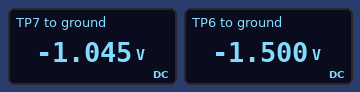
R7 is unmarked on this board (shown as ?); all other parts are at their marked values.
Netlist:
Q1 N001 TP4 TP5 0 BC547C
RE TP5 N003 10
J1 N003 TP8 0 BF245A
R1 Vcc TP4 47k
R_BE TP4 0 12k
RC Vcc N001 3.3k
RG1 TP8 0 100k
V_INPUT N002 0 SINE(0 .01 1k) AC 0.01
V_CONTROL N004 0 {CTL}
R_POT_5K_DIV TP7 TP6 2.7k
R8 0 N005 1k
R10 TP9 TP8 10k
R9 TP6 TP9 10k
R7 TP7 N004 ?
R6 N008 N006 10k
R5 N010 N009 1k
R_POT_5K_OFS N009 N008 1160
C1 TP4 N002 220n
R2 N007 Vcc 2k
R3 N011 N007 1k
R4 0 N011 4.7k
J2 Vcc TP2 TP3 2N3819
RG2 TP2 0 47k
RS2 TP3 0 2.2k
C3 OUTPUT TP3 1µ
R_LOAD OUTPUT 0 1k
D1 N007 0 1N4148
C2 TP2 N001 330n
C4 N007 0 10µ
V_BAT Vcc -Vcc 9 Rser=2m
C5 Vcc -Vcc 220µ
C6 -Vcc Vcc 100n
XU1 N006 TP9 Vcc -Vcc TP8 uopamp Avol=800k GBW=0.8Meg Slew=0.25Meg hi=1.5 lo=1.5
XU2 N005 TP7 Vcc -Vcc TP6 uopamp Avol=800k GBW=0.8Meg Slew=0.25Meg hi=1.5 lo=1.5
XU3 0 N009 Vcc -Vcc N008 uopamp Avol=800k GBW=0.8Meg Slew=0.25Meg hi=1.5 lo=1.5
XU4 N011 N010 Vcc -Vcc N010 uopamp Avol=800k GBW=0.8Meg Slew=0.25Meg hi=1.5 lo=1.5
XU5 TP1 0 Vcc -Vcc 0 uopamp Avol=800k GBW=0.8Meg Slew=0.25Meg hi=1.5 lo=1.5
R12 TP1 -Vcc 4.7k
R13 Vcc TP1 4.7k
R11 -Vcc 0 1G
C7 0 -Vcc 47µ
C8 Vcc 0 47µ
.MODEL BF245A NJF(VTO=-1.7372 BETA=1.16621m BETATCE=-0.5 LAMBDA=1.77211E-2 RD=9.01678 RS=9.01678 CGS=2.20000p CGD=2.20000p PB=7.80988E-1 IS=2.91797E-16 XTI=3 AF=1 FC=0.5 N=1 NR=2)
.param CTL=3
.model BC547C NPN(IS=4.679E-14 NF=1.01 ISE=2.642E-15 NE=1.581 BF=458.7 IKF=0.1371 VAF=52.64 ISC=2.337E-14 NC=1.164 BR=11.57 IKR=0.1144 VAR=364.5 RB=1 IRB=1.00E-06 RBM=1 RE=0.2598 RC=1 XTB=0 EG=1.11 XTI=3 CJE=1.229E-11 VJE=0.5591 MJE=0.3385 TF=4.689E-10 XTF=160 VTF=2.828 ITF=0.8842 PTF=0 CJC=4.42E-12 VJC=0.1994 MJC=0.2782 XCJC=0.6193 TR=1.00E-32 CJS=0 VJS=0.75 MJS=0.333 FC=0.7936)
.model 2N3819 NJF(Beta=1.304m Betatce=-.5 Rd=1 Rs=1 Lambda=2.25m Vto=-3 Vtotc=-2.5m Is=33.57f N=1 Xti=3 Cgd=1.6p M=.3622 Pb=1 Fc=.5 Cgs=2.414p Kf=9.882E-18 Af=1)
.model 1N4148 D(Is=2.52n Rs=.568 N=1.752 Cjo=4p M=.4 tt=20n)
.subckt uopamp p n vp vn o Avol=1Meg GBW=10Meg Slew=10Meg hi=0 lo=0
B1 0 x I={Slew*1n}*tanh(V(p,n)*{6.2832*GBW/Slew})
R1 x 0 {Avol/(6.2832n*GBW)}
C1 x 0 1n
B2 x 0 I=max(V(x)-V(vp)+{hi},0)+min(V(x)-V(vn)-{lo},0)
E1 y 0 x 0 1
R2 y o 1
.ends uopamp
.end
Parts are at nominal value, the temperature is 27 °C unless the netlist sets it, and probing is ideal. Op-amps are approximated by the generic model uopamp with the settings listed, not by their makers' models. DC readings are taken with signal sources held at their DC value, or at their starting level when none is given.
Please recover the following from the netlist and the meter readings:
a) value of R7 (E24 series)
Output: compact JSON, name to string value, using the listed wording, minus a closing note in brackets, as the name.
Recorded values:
{"value of R7": "24 kΩ"}
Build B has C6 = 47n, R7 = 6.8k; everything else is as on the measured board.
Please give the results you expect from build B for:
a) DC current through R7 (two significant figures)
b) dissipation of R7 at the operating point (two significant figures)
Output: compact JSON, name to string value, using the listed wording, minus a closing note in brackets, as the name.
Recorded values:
{"DC current through R7": "470 µA", "dissipation of R7 at the operating point": "1.5 mW"}
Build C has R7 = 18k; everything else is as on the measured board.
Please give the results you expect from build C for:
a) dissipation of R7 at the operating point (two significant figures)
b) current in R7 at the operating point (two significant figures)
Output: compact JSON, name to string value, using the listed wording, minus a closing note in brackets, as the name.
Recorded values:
{"dissipation of R7 at the operating point": "850 µW", "current in R7 at the operating point": "220 µA"}
